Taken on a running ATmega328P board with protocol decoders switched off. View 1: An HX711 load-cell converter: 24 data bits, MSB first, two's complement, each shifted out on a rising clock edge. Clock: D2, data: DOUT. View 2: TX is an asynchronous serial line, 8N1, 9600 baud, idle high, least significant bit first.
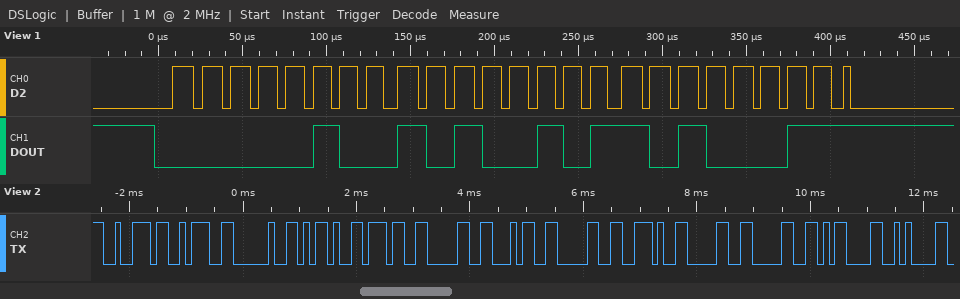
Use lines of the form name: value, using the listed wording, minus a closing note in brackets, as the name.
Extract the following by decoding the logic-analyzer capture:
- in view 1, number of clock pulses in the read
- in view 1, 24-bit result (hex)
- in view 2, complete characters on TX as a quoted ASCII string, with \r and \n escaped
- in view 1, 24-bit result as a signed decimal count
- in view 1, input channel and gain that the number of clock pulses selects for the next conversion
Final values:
in view 1, number of clock pulses in the read: 25
in view 1, 24-bit result: 0x04A5A3
in view 2, complete characters on TX as a quoted ASCII string, with \r and \n escaped: "r: -7040.00\r\n"
in view 1, 24-bit result as a signed decimal count: 304547
in view 1, input channel and gain that the number of clock pulses selects for the next conversion: channel A, gain 128
